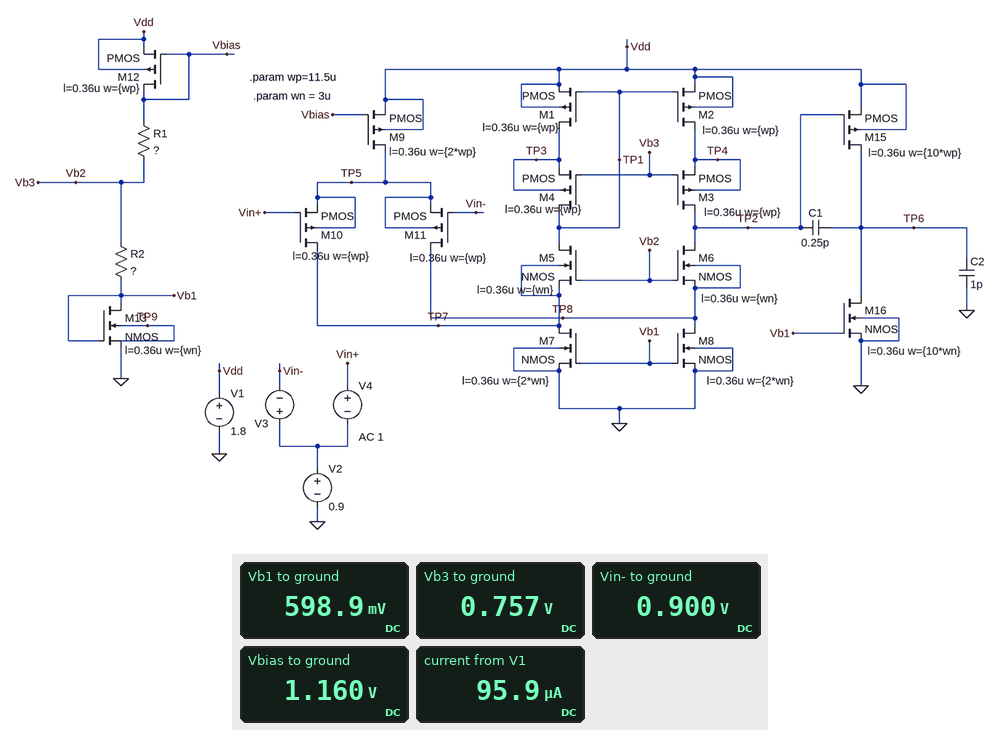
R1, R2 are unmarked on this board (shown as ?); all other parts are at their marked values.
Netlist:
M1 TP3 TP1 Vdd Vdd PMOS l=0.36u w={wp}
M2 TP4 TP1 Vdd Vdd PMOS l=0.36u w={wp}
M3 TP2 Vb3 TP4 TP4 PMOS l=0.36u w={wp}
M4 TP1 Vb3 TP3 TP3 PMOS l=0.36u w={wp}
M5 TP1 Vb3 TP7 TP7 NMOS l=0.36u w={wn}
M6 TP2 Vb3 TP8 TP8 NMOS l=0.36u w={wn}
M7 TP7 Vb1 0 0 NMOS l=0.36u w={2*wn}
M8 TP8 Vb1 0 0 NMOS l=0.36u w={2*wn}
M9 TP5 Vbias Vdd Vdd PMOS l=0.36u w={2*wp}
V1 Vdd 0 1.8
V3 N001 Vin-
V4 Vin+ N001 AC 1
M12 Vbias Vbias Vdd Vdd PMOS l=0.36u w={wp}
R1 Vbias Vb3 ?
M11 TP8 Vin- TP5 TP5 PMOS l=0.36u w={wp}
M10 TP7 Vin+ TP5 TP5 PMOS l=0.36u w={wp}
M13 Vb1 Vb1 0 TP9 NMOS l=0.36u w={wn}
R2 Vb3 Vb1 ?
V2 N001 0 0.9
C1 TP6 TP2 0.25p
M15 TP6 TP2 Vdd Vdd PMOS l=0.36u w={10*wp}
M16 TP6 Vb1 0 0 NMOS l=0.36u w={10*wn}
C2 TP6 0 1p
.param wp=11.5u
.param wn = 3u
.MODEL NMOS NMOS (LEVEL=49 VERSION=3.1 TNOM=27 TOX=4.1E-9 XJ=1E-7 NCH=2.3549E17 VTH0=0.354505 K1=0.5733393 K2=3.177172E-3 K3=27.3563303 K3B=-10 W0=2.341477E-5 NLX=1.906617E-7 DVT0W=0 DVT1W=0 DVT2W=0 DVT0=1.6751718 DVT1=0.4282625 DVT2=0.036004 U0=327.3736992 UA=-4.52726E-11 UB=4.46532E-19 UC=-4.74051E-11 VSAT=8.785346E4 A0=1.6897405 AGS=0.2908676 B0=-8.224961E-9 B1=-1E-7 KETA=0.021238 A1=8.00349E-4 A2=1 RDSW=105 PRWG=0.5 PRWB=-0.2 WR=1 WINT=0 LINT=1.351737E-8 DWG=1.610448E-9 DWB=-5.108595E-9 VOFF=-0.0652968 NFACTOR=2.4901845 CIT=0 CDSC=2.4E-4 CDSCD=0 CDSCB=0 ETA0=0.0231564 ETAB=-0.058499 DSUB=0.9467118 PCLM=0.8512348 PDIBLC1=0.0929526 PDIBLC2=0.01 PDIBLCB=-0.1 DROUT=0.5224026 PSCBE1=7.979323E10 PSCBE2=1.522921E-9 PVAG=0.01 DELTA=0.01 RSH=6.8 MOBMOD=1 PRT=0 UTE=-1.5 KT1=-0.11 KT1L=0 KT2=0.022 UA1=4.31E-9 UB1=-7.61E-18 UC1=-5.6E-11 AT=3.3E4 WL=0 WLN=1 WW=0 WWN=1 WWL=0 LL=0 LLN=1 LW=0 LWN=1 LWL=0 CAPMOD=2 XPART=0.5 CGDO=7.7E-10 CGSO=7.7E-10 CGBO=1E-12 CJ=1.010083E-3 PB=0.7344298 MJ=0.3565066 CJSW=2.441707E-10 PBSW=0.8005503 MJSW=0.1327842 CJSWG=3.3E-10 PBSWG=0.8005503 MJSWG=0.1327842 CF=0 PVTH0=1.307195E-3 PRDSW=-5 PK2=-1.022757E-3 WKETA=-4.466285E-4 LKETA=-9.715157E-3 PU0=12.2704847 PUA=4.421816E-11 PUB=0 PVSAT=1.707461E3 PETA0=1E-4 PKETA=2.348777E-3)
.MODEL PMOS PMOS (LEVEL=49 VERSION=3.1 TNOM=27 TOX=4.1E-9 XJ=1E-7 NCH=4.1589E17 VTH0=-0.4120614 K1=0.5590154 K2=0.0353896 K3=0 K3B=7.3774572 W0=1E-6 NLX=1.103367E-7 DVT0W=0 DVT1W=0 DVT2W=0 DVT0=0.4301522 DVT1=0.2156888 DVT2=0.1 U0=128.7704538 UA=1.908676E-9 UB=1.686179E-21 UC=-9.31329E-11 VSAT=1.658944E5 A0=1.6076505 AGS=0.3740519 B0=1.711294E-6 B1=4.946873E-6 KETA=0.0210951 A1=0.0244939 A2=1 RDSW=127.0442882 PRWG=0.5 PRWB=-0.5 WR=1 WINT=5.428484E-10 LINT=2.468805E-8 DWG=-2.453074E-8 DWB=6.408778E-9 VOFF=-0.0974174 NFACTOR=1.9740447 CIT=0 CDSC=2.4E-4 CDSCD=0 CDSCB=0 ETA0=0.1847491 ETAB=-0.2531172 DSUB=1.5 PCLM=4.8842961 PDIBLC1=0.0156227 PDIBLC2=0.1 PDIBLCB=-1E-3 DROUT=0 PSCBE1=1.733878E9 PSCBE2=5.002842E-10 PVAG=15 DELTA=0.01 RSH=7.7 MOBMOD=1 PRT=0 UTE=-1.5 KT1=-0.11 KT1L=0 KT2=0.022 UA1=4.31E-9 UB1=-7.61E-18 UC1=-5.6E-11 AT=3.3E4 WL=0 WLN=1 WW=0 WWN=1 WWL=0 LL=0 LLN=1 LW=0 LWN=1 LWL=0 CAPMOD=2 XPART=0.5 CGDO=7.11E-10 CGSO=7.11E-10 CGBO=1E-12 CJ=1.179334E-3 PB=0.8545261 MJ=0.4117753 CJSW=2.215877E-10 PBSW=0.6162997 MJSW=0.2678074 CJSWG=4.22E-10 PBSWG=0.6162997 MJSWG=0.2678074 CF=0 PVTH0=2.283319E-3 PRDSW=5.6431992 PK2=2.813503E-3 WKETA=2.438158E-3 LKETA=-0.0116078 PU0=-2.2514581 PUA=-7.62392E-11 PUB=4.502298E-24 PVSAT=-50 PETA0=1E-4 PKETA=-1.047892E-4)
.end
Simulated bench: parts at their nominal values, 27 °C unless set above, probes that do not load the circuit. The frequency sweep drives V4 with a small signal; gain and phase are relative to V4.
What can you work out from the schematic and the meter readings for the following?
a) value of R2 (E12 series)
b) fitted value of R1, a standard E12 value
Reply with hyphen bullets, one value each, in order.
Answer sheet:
- 4.7 kΩ
- 12 kΩ
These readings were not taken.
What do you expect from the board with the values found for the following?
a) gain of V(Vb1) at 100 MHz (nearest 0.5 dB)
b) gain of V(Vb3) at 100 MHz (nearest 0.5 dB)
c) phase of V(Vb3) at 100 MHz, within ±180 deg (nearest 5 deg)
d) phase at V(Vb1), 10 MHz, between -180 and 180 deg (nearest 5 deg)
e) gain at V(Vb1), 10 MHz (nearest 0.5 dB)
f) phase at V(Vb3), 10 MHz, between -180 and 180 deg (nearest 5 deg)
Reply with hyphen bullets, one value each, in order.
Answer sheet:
- -47.0 dB
- -40.0 dB
- 115 deg
- -125 deg
- -68.5 dB
- -125 deg
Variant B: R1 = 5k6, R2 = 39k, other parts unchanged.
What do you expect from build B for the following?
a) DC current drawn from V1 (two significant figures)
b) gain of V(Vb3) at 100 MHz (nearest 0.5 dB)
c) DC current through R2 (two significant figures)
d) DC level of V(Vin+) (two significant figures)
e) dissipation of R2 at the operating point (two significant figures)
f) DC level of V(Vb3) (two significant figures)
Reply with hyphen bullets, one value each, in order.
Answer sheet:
- 40 µA
- -36.5 dB
- 15 µA
- 900 mV
- 9.0 µW
- 1.1 V
